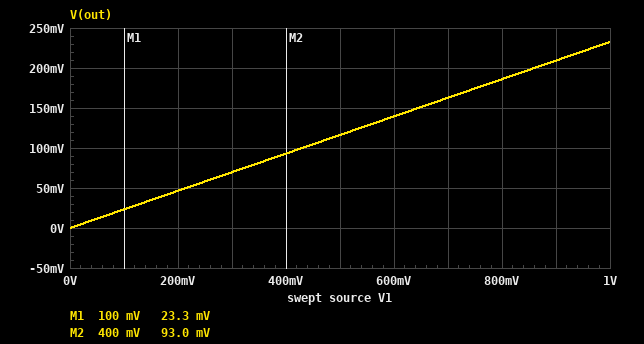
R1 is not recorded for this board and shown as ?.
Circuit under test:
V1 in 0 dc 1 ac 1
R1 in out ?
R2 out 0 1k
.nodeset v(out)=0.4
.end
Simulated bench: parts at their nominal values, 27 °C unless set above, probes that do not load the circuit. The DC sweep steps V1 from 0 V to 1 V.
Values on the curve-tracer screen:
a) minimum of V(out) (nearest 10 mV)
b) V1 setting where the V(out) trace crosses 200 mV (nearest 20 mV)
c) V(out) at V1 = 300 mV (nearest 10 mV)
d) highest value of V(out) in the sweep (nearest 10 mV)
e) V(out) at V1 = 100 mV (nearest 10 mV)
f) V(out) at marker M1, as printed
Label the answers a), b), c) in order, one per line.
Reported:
a) 0 V
b) 860 mV
c) 70 mV
d) 230 mV
e) 20 mV
f) 23.3 mV
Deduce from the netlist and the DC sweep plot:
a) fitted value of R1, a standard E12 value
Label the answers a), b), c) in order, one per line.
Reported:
a) 3.3 kΩ
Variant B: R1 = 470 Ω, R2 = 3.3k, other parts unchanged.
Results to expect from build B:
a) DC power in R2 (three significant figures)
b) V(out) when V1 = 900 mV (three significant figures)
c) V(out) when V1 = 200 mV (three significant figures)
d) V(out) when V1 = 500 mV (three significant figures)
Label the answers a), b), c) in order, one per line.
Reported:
a) 232 µW
b) 788 mV
c) 175 mV
d) 438 mV
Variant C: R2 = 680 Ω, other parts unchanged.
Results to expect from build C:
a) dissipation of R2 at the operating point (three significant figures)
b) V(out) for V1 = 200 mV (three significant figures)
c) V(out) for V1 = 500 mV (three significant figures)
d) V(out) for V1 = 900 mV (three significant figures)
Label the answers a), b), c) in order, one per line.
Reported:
a) 42.9 µW
b) 34.2 mV
c) 85.4 mV
d) 154 mV
